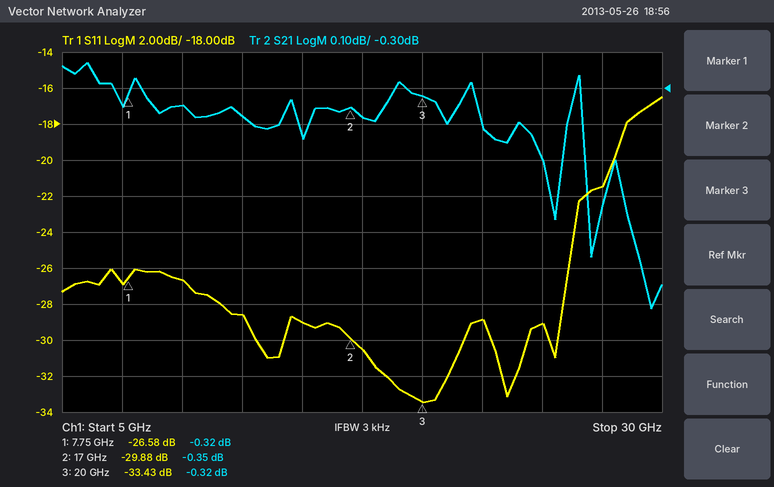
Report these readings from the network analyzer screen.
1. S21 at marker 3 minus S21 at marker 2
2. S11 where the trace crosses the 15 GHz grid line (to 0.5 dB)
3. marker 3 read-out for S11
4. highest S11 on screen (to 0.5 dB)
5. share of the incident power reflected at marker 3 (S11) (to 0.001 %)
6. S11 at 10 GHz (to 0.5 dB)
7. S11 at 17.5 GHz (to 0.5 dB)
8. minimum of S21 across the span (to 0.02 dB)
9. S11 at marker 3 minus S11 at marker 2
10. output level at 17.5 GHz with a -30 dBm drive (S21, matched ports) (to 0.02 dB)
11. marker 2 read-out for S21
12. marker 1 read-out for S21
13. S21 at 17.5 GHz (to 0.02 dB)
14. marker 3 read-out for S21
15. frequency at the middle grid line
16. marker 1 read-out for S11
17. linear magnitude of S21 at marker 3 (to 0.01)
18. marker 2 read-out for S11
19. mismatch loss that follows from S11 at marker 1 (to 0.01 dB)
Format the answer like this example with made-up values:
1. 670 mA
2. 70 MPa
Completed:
1. 0.03 dB
2. -29.0 dB
3. -33.43 dB
4. -16.5 dB
5. 0.045 %
6. -26.5 dB
7. -30.5 dB
8. -0.92 dB
9. -3.55 dB
10. -30.38 dBm
11. -0.35 dB
12. -0.32 dB
13. -0.38 dB
14. -0.32 dB
15. 17.5 GHz
16. -26.58 dB
17. 0.96
18. -29.88 dB
19. 0.01 dB
